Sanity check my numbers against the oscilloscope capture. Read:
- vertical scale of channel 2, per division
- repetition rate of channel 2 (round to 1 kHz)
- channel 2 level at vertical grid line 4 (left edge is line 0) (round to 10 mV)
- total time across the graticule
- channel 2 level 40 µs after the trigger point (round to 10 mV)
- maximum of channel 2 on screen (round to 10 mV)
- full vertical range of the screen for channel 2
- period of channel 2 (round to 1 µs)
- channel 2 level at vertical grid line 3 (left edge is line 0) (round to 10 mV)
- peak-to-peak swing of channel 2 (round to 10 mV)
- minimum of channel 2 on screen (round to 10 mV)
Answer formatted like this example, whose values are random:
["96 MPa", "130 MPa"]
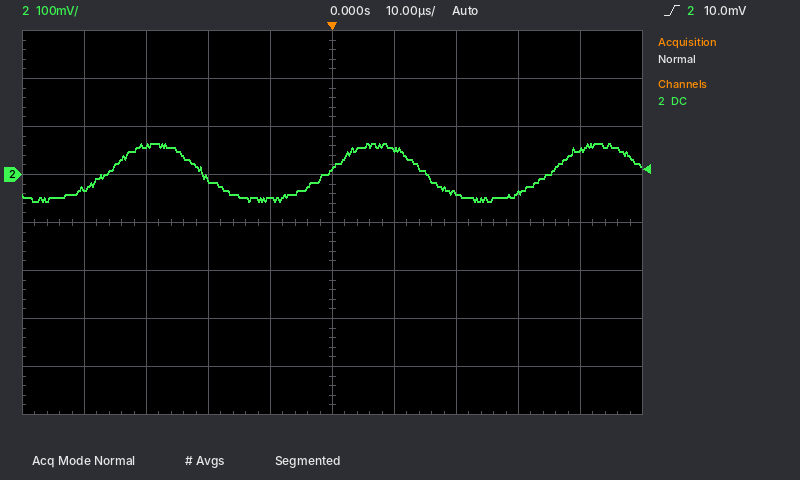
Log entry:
["100 mV", "28 kHz", "-50 mV", "100 µs", "50 mV", "60 mV", "800 mV", "36 µs", "-10 mV", "120 mV", "-60 mV"]
